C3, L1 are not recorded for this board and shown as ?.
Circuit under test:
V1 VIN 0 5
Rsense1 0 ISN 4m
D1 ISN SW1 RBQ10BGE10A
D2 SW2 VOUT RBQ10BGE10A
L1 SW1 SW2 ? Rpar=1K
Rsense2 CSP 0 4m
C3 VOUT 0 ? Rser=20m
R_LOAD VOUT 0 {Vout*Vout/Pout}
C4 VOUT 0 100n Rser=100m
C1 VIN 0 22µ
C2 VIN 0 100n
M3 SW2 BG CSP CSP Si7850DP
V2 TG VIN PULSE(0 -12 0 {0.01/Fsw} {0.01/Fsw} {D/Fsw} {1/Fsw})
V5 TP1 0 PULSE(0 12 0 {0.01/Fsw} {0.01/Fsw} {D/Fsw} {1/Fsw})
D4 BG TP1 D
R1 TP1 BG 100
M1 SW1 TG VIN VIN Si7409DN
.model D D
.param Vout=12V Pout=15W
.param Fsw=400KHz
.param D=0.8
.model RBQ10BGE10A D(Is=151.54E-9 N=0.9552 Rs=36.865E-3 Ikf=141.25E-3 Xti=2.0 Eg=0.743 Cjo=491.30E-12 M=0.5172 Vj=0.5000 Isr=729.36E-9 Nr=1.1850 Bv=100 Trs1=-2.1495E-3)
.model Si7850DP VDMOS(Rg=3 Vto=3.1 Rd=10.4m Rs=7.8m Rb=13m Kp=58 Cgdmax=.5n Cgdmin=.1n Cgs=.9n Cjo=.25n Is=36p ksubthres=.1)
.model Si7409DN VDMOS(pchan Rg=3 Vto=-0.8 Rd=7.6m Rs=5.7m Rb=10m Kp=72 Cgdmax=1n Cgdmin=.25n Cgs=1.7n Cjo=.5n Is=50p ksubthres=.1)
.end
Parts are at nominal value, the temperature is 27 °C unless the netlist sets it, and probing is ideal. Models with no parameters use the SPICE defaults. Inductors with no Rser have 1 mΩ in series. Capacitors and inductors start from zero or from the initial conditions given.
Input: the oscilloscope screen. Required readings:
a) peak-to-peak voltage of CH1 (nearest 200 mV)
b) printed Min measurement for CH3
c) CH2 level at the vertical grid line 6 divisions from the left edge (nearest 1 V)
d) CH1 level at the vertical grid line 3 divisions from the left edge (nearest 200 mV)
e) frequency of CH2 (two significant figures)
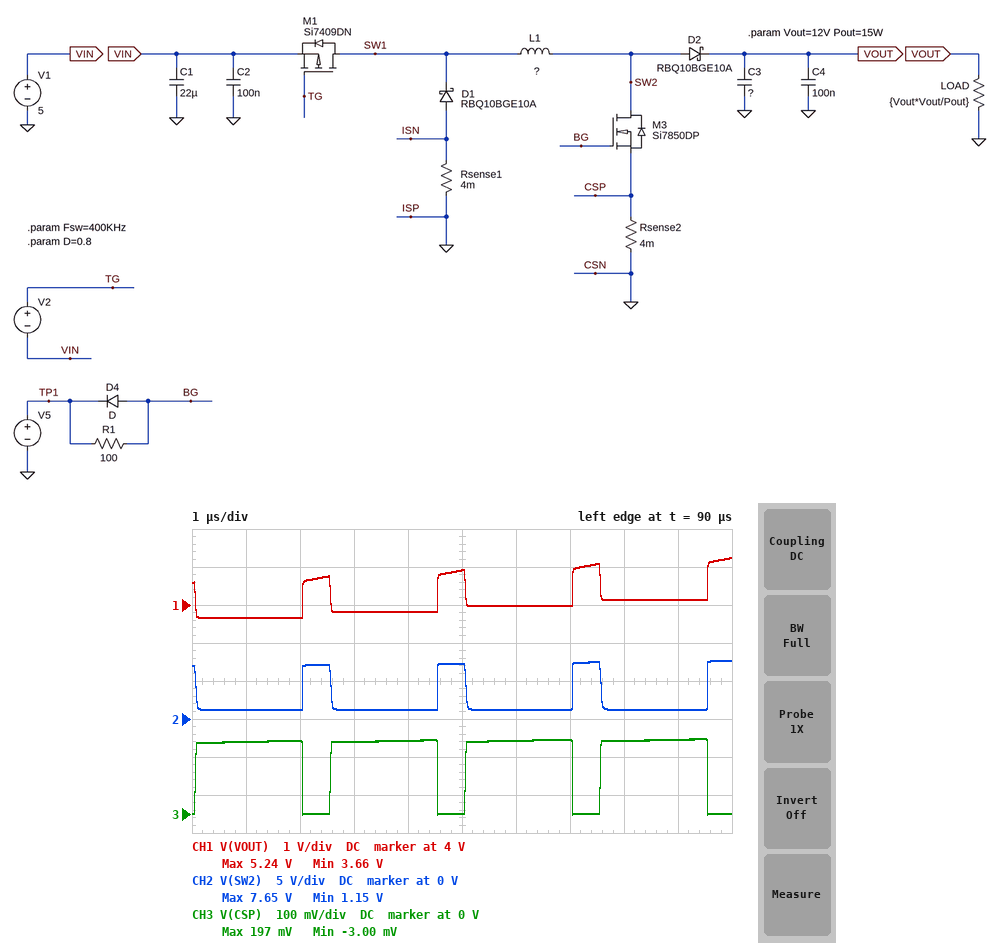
1.6 V
-3.00 mV
1 V
3.8 V
400 kHz
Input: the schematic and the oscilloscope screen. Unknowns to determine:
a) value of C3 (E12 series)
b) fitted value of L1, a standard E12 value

150 µF
3.9 µH
